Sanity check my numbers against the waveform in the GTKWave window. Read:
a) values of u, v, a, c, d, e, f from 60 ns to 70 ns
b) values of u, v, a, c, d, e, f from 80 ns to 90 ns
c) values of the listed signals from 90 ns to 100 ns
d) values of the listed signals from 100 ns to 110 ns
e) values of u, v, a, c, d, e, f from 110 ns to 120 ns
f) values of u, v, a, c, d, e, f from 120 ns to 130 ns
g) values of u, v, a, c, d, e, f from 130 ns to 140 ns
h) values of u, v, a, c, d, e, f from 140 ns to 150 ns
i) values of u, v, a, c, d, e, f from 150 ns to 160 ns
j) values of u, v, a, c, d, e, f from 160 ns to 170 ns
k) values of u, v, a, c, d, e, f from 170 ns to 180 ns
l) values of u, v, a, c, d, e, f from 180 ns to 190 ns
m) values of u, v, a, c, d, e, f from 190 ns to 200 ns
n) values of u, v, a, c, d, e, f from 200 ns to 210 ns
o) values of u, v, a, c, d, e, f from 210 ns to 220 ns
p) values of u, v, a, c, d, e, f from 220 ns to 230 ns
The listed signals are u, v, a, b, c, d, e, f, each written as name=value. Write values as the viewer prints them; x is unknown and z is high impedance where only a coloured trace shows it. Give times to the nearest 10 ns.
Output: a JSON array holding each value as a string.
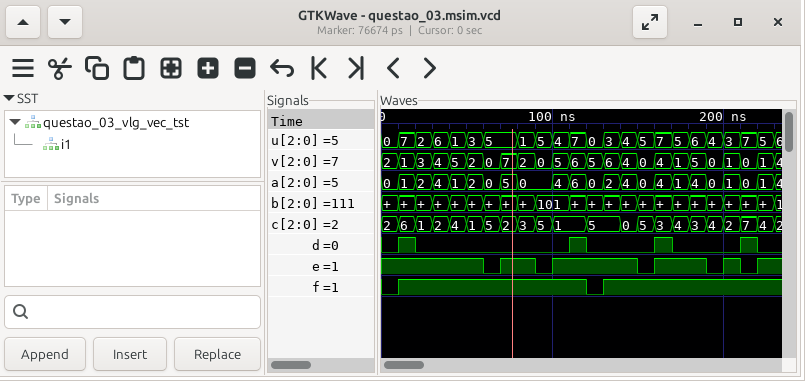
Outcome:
["u=5, v=0, a=0, c=5, d=0, e=0, f=1", "u=1, v=2, a=0, c=3, d=0, e=1, f=1", "u=5, v=0, a=0, b=101, c=5, d=0, e=0, f=1", "u=4, v=5, a=4, b=101, c=1, d=0, e=1, f=1", "u=7, v=6, a=6, c=1, d=1, e=1, f=1", "u=0, v=5, a=0, c=5, d=0, e=1, f=0", "u=3, v=6, a=2, c=5, d=0, e=1, f=1", "u=4, v=4, a=4, c=0, d=0, e=1, f=1", "u=5, v=0, a=0, c=5, d=0, e=0, f=1", "u=7, v=4, a=4, c=3, d=1, e=1, f=1", "u=5, v=1, a=1, c=4, d=0, e=1, f=1", "u=6, v=5, a=4, c=3, d=0, e=1, f=1", "u=4, v=0, a=0, c=4, d=0, e=0, f=1", "u=3, v=1, a=1, c=2, d=0, e=1, f=1", "u=7, v=0, a=0, c=7, d=1, e=0, f=1", "u=5, v=1, a=1, c=4, d=0, e=1, f=1"]
